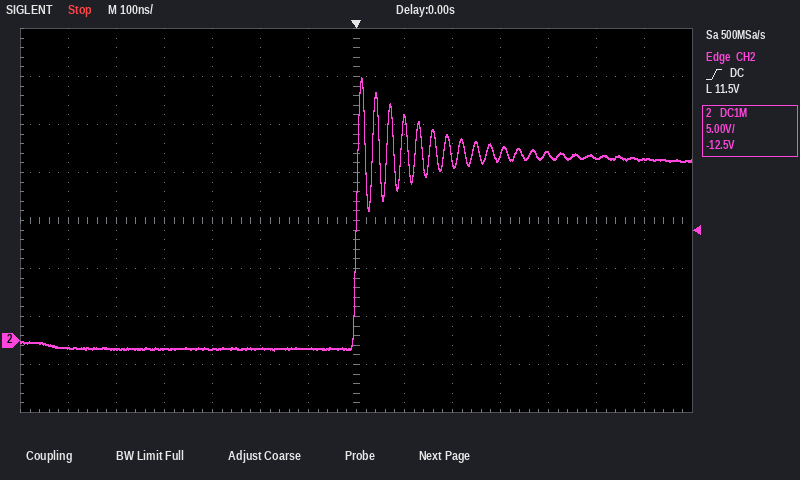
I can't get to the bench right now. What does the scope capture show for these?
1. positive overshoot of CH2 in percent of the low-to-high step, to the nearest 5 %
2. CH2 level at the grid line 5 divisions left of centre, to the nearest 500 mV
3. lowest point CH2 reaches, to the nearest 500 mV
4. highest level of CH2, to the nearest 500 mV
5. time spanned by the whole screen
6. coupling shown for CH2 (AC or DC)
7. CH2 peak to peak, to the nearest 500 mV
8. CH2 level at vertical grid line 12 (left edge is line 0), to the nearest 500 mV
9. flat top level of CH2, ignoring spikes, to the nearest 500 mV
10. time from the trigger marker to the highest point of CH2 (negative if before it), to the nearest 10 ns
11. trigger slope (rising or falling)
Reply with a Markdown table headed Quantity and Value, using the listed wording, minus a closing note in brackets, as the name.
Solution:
| Quantity | Value |
|---|---|
| positive overshoot of CH2 in percent of the low-to-high step, to the nearest 5 % | 45 % |
| CH2 level at the grid line 5 divisions left of centre, to the nearest 500 mV | -1.0 V |
| lowest point CH2 reaches, to the nearest 500 mV | -1.0 V |
| highest level of CH2, to the nearest 500 mV | 27.5 V |
| time spanned by the whole screen | 1.4 µs |
| coupling shown for CH2 | DC |
| CH2 peak to peak, to the nearest 500 mV | 28.5 V |
| CH2 level at vertical grid line 12 (left edge is line 0), to the nearest 500 mV | 19.0 V |
| flat top level of CH2, ignoring spikes, to the nearest 500 mV | 19.0 V |
| time from the trigger marker to the highest point of CH2 (negative if before it), to the nearest 10 ns | +10 ns |
| trigger slope | rising |
